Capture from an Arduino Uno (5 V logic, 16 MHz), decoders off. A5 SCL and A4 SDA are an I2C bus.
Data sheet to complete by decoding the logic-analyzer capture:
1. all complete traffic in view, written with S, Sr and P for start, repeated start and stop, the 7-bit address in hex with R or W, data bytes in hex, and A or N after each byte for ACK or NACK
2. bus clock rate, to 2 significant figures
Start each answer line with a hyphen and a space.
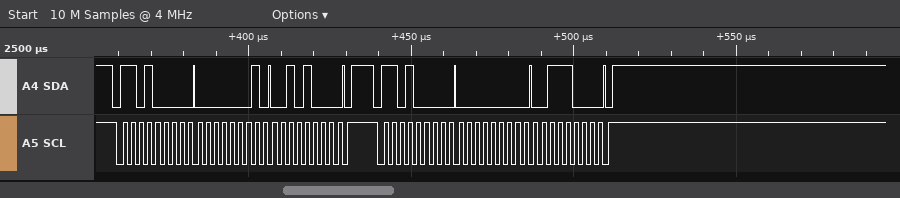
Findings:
- S 68W A 01 A 28 A P S 68W A 00 A 38 A P
- 400 kHz
